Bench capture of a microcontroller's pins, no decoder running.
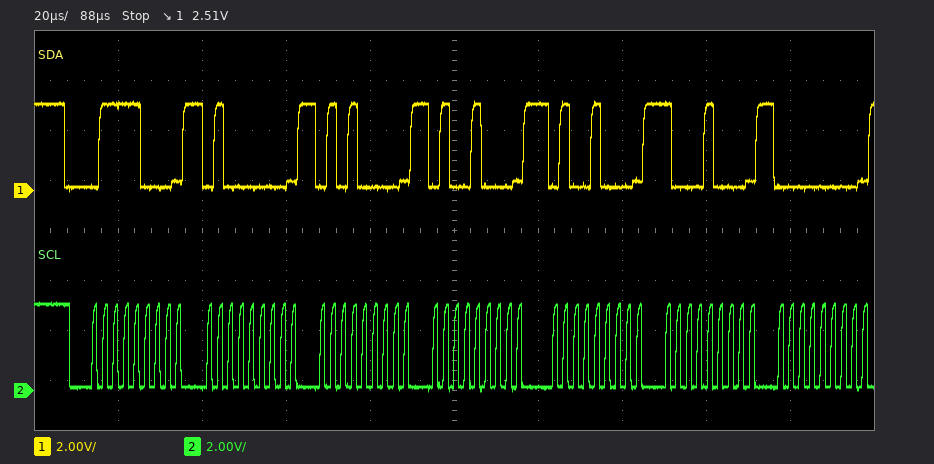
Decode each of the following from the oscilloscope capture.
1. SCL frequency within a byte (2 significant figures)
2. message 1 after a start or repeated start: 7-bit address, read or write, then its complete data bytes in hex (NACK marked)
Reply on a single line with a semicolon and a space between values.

400 kHz; 0x3C write: 40 50 48 48 88 00
